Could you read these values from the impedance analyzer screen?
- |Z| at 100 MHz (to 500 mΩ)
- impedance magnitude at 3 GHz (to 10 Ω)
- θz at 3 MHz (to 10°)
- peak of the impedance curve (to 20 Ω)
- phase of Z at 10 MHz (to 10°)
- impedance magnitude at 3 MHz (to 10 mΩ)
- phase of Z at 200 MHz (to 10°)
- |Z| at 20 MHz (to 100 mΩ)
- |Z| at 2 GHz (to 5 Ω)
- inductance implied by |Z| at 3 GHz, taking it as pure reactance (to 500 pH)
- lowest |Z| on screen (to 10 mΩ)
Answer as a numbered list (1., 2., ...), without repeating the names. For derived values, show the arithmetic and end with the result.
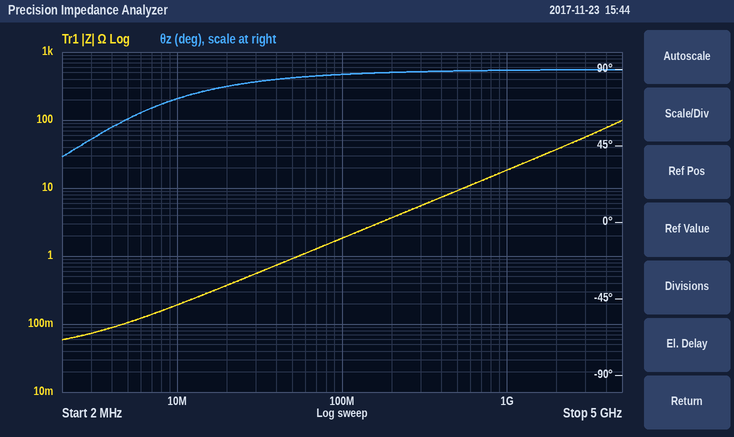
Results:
1. 2.0 Ω
2. 60 Ω
3. 50°
4. 100 Ω
5. 70°
6. 70 mΩ
7. 90°
8. 400 mΩ
9. 35 Ω
10. L = 60 Ω/(2π × 3 GHz) ≈ 3.18 nH, so 3.0 nH to the nearest 500 pH
11. 60 mΩ
